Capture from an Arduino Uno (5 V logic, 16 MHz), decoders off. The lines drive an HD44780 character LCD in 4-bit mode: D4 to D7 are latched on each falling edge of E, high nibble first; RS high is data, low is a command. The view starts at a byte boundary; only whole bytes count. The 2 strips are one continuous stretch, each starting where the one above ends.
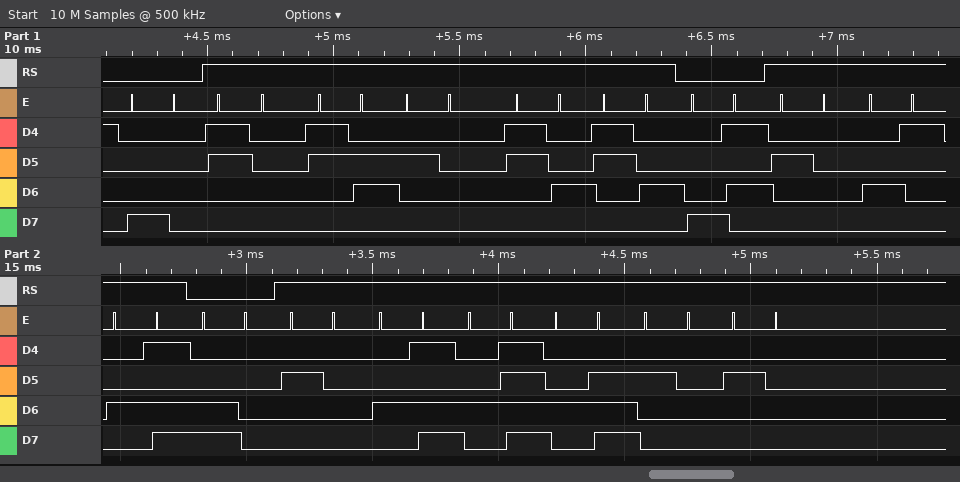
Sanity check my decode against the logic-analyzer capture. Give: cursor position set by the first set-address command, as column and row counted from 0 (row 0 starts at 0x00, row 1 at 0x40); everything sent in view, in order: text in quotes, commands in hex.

column 0, row 0
0x80 "06 44" 0x85 " AM" 0xC0 " MON  "
